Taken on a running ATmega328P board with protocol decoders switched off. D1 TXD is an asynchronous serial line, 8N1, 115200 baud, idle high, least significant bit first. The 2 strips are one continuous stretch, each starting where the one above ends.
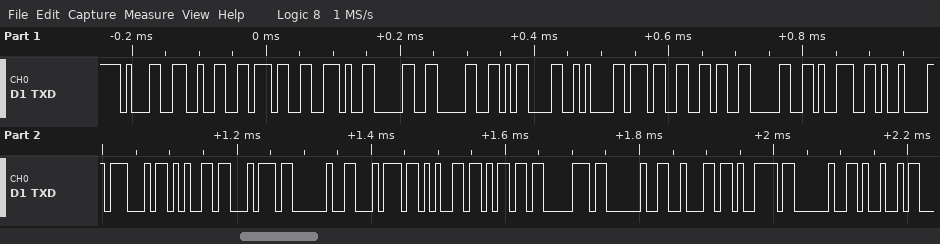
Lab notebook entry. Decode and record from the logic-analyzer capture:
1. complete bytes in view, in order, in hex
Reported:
31 32 37 2E 30 30 0D 0A 37 36 30 39 09 47 65 74 20 74 65 6D 70 20 62 79 20 49
